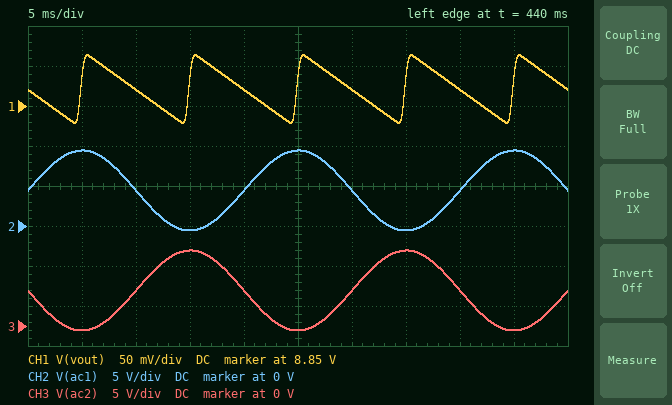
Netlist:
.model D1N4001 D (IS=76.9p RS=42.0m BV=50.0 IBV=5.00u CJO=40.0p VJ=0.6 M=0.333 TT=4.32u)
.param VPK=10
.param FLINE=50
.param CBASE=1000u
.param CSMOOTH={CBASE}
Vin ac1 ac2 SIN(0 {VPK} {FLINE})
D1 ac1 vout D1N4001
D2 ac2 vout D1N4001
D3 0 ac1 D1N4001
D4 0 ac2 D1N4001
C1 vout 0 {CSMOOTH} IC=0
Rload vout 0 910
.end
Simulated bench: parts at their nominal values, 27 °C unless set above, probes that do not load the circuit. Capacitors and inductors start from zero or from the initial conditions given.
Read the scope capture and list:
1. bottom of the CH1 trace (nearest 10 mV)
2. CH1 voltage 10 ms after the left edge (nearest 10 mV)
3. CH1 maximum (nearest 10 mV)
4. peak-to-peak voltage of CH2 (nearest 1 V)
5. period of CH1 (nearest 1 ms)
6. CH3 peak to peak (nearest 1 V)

8.83 V
8.87 V
8.91 V
10 V
10 ms
10 V
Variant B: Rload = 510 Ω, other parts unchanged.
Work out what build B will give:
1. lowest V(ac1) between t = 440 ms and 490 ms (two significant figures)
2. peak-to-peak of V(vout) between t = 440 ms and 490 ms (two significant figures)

-580 mV
150 mV
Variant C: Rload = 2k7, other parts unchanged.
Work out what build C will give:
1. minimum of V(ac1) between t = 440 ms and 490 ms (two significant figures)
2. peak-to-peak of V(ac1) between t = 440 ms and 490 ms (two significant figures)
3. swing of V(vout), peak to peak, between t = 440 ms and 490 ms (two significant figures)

-530 mV
10 V
29 mV
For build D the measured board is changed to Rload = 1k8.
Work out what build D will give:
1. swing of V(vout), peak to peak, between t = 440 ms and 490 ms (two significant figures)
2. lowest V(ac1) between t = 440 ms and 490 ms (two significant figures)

43 mV
-540 mV
